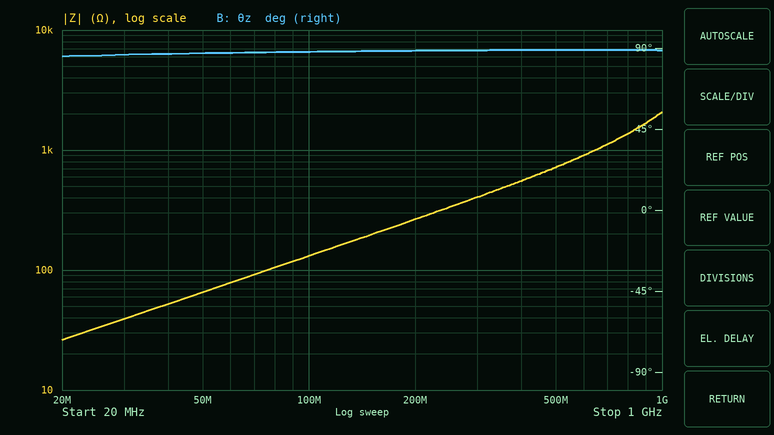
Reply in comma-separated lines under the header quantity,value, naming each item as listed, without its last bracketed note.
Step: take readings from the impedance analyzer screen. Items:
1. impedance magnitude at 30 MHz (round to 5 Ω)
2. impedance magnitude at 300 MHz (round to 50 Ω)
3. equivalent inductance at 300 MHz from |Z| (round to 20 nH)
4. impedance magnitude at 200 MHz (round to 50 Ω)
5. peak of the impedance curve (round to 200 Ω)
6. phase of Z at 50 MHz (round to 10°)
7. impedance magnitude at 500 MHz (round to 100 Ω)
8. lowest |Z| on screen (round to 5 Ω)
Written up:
quantity,value
impedance magnitude at 30 MHz,40 Ω
impedance magnitude at 300 MHz,400 Ω
equivalent inductance at 300 MHz from |Z|,220 nH
impedance magnitude at 200 MHz,250 Ω
peak of the impedance curve,2.0 kΩ
phase of Z at 50 MHz,90°
impedance magnitude at 500 MHz,700 Ω
lowest |Z| on screen,25 Ω
